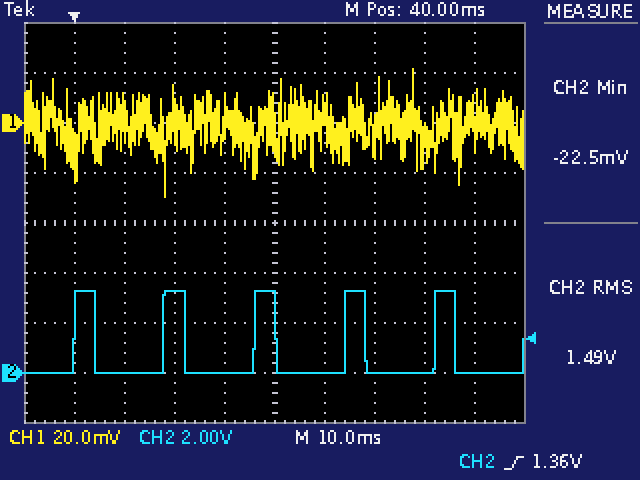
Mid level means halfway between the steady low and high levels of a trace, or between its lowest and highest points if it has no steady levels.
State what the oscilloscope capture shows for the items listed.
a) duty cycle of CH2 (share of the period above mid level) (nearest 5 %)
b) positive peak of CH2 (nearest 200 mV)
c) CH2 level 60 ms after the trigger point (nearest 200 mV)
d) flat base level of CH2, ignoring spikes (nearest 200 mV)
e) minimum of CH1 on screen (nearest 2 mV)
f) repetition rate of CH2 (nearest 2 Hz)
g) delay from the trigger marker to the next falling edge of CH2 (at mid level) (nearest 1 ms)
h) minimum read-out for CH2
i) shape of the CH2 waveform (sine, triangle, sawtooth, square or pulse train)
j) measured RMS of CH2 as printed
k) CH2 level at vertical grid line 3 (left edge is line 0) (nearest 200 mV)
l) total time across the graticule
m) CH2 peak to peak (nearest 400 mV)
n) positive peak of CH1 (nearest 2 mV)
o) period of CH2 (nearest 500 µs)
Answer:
25 %
3.2 V
0.0 V
0.0 V
-30 mV
56 Hz
4 ms
-22.5 mV
pulse train
1.49 V
3.2 V
100 ms
3.2 V
22 mV
18.0 ms
